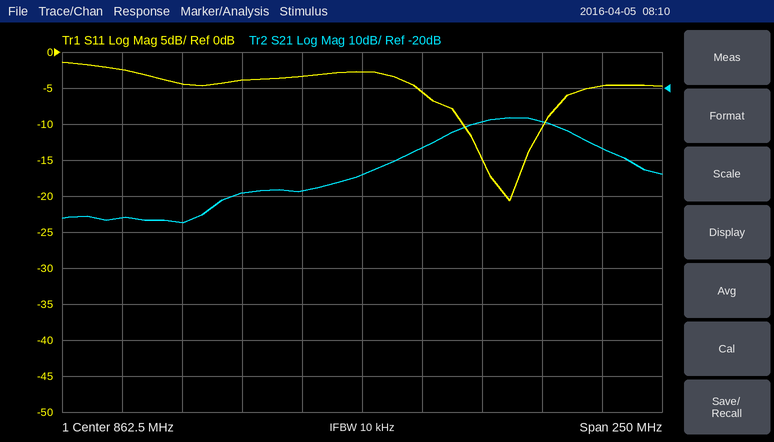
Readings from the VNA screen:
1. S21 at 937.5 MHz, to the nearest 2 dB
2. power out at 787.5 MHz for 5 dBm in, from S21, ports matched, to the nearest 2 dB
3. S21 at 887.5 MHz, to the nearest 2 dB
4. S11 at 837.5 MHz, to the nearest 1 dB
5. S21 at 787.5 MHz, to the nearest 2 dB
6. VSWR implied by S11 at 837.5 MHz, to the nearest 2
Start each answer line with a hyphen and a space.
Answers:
- -30 dB
- -52 dBm
- -36 dB
- -3 dB
- -58 dB
- 6
